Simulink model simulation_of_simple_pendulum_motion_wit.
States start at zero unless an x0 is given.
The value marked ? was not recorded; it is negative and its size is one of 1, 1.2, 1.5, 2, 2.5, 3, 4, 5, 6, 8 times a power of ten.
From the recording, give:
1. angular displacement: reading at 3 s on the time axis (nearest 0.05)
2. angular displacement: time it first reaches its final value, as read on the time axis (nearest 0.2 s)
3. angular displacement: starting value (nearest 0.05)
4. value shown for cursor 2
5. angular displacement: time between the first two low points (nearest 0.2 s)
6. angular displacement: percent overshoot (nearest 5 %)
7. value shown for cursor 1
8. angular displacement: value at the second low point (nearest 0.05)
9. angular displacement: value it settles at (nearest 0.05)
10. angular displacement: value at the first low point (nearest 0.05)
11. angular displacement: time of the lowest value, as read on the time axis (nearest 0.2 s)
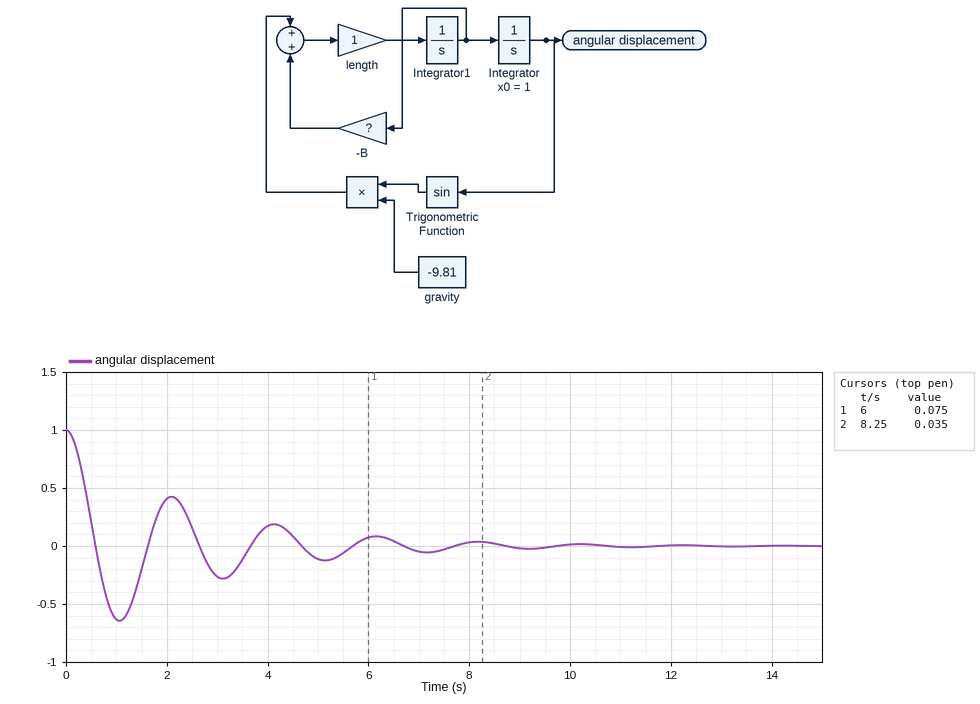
-0.25
0.6 s
1.00
0.035
2.0 s
65 %
0.075
-0.30
0.00
-0.65
1.0 s
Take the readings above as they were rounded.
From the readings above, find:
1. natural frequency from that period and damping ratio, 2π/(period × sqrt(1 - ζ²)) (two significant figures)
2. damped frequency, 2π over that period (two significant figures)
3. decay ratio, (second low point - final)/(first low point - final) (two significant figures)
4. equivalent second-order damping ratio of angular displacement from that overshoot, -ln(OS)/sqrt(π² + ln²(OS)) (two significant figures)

3.2 rad/s
3.1 rad/s
0.46
0.14
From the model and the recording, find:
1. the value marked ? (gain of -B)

-0.8
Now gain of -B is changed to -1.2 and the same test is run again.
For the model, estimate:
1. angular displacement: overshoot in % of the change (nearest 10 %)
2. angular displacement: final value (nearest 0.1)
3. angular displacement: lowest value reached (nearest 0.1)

50 %
0.0
-0.5
